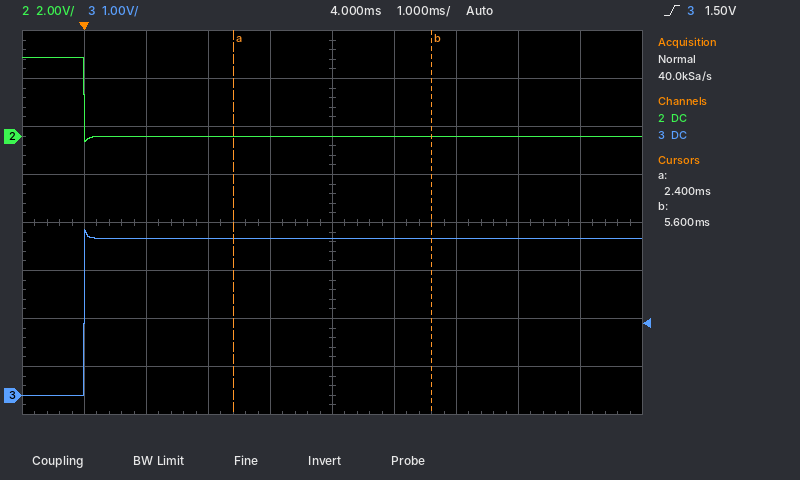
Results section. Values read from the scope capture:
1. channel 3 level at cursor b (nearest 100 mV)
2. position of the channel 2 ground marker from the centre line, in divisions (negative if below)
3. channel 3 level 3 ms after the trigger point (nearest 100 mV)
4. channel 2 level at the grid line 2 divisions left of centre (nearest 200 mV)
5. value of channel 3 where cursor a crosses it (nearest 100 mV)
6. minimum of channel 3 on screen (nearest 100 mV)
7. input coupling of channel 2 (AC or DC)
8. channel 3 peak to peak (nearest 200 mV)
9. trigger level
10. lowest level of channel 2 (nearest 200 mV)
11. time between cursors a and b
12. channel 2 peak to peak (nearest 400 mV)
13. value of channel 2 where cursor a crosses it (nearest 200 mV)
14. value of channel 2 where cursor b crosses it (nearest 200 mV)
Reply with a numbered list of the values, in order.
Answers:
1. 3.3 V
2. +1.8 div
3. 3.3 V
4. 0.0 V
5. 3.3 V
6. 0.0 V
7. DC
8. 3.4 V
9. 1.50 V
10. -200 mV
11. 3.2 ms
12. 3.6 V
13. 0.0 V
14. 0.0 V
